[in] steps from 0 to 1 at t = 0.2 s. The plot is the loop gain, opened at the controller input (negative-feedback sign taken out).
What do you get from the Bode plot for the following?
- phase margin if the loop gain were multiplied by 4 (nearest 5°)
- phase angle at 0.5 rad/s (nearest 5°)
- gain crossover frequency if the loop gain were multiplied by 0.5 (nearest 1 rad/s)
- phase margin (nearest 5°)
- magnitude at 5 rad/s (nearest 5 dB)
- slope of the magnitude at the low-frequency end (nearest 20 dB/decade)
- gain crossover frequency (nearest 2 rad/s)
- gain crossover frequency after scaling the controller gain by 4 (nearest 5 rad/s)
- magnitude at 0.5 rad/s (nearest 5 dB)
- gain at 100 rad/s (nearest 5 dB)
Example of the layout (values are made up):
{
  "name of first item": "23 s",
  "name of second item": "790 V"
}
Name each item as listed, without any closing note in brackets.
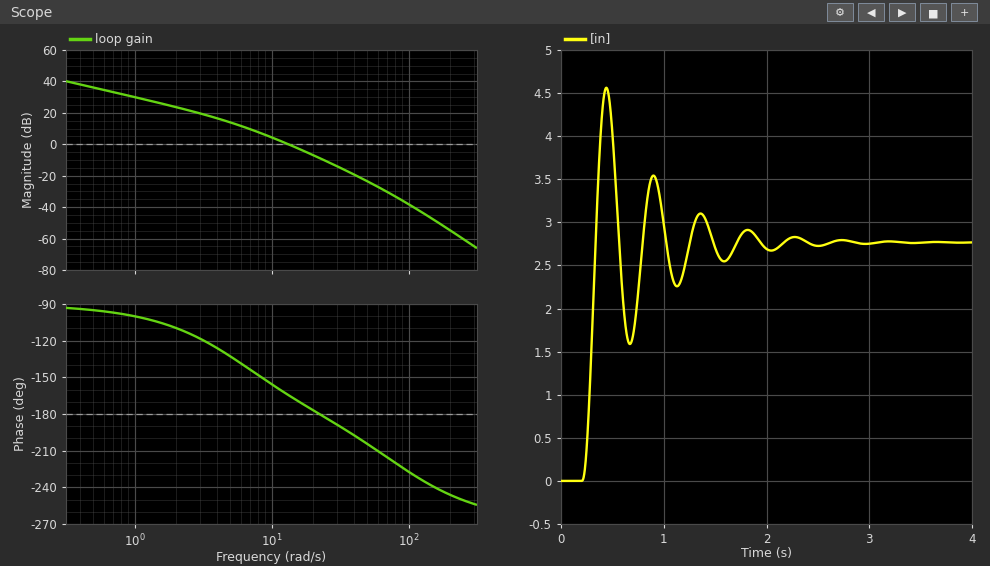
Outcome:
{
  "phase margin if the loop gain were multiplied by 4": "-5°",
  "phase angle at 0.5 rad/s": "-95°",
  "gain crossover frequency if the loop gain were multiplied by 0.5": "9 rad/s",
  "phase margin": "15°",
  "magnitude at 5 rad/s": "15 dB",
  "slope of the magnitude at the low-frequency end": "-20 dB/decade",
  "gain crossover frequency": "14 rad/s",
  "gain crossover frequency after scaling the controller gain by 4": "25 rad/s",
  "magnitude at 0.5 rad/s": "35 dB",
  "gain at 100 rad/s": "-40 dB"
}
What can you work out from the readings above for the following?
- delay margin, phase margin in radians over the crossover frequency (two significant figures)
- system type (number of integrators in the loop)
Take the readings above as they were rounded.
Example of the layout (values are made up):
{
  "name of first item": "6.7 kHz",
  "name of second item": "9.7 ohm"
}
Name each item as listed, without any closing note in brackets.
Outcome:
{
  "delay margin, phase margin in radians over the crossover frequency": "0.019 s",
  "system type": "1"
}
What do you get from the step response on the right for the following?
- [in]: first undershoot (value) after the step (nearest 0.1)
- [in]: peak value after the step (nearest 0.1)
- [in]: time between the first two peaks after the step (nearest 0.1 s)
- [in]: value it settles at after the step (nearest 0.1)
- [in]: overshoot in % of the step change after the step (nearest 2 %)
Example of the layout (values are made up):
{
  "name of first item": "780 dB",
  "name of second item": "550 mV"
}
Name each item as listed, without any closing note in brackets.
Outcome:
{
  "[in]: first undershoot (value) after the step": "1.6",
  "[in]: peak value after the step": "4.6",
  "[in]: time between the first two peaks after the step": "0.5 s",
  "[in]: value it settles at after the step": "2.8",
  "[in]: overshoot in % of the step change after the step": "64 %"
}
